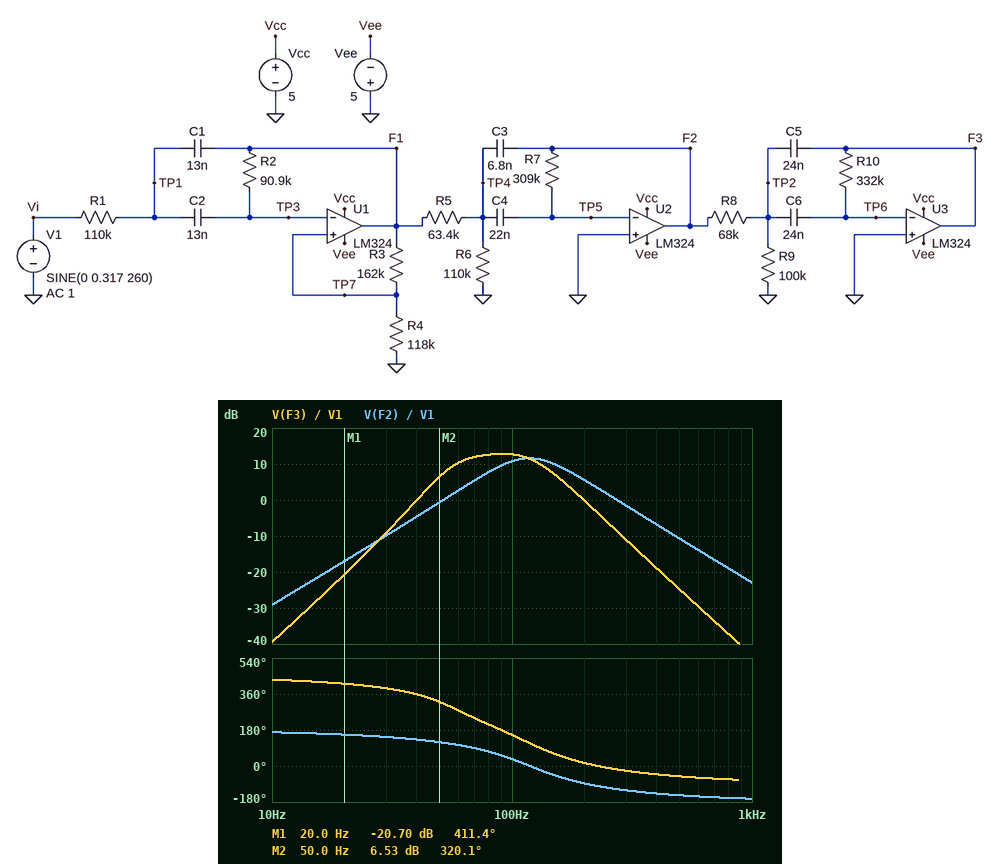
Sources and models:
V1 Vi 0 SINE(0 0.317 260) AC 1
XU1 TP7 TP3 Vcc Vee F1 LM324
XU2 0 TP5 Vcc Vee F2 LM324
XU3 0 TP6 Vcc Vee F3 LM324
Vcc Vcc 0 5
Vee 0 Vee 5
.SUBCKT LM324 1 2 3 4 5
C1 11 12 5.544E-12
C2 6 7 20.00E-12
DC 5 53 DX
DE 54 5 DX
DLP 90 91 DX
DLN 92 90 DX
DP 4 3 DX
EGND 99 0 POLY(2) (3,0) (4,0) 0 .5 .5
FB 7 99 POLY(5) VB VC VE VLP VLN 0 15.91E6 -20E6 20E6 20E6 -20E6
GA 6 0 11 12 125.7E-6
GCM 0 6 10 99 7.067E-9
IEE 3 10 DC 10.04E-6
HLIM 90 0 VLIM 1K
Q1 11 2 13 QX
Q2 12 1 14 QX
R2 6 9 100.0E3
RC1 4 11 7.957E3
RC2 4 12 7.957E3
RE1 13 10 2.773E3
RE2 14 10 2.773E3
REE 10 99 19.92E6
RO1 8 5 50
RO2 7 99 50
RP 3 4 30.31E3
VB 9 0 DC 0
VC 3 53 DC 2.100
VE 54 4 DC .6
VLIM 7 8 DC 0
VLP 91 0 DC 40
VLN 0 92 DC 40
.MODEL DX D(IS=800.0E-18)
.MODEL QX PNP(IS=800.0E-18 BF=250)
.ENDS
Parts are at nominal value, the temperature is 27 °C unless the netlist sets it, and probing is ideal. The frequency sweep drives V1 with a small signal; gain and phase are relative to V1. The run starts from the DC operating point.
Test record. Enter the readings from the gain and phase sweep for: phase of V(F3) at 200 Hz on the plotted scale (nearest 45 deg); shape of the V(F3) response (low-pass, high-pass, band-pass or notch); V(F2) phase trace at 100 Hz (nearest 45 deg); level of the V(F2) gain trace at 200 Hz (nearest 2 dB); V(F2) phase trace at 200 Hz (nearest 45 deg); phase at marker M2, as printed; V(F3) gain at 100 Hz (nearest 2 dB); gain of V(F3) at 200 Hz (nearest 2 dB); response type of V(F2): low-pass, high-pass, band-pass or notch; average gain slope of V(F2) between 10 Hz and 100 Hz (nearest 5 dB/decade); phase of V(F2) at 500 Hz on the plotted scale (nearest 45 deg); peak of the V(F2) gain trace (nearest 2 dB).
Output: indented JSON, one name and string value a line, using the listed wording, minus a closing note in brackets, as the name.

{
  "phase of V(F3) at 200 Hz on the plotted scale": "0 deg",
  "shape of the V(F3) response": "band-pass",
  "V(F2) phase trace at 100 Hz": "45 deg",
  "level of the V(F2) gain trace at 200 Hz": "6 dB",
  "V(F2) phase trace at 200 Hz": "-90 deg",
  "phase at marker M2, as printed": "320.1 deg",
  "V(F3) gain at 100 Hz": "12 dB",
  "gain of V(F3) at 200 Hz": "0 dB",
  "response type of V(F2): low-pass, high-pass, band-pass or notch": "band-pass",
  "average gain slope of V(F2) between 10 Hz and 100 Hz": "40 dB/decade",
  "phase of V(F2) at 500 Hz on the plotted scale": "-135 deg",
  "peak of the V(F2) gain trace": "12 dB"
}
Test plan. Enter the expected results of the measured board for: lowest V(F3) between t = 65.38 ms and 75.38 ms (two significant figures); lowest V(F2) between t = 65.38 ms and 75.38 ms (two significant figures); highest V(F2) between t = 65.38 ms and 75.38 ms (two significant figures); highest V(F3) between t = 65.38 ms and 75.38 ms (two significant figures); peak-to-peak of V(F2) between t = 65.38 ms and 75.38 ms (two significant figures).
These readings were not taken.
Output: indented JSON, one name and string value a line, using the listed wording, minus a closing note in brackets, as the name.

{
  "lowest V(F3) between t = 65.38 ms and 75.38 ms": "-140 mV",
  "lowest V(F2) between t = 65.38 ms and 75.38 ms": "-360 mV",
  "highest V(F2) between t = 65.38 ms and 75.38 ms": "350 mV",
  "highest V(F3) between t = 65.38 ms and 75.38 ms": "130 mV",
  "peak-to-peak of V(F2) between t = 65.38 ms and 75.38 ms": "710 mV"
}
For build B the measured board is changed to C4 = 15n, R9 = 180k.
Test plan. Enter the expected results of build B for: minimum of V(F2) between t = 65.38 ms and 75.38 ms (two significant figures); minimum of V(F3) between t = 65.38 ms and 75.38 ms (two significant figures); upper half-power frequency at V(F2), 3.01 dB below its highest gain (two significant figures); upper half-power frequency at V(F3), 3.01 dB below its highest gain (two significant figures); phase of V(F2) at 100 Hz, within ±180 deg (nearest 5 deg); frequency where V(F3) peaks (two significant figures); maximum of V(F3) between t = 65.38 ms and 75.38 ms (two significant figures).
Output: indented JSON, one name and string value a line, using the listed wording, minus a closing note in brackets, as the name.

{
  "minimum of V(F2) between t = 65.38 ms and 75.38 ms": "-390 mV",
  "minimum of V(F3) between t = 65.38 ms and 75.38 ms": "-150 mV",
  "upper half-power frequency at V(F2), 3.01 dB below its highest gain": "190 Hz",
  "upper half-power frequency at V(F3), 3.01 dB below its highest gain": "160 Hz",
  "phase of V(F2) at 100 Hz, within ±180 deg": "55 deg",
  "frequency where V(F3) peaks": "110 Hz",
  "maximum of V(F3) between t = 65.38 ms and 75.38 ms": "140 mV"
}
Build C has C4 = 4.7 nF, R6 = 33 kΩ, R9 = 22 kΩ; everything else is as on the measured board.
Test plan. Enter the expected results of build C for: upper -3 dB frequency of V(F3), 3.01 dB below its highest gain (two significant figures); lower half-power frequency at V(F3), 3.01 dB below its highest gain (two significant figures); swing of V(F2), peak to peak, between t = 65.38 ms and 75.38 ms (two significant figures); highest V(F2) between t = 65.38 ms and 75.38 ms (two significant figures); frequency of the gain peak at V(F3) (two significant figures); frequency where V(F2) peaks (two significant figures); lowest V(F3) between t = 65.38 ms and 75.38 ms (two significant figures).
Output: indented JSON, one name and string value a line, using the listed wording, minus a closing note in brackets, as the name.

{
  "upper -3 dB frequency of V(F3), 3.01 dB below its highest gain": "150 Hz",
  "lower half-power frequency at V(F3), 3.01 dB below its highest gain": "80 Hz",
  "swing of V(F2), peak to peak, between t = 65.38 ms and 75.38 ms": "610 mV",
  "highest V(F2) between t = 65.38 ms and 75.38 ms": "300 mV",
  "frequency of the gain peak at V(F3)": "97 Hz",
  "frequency where V(F2) peaks": "320 Hz",
  "lowest V(F3) between t = 65.38 ms and 75.38 ms": "-130 mV"
}
